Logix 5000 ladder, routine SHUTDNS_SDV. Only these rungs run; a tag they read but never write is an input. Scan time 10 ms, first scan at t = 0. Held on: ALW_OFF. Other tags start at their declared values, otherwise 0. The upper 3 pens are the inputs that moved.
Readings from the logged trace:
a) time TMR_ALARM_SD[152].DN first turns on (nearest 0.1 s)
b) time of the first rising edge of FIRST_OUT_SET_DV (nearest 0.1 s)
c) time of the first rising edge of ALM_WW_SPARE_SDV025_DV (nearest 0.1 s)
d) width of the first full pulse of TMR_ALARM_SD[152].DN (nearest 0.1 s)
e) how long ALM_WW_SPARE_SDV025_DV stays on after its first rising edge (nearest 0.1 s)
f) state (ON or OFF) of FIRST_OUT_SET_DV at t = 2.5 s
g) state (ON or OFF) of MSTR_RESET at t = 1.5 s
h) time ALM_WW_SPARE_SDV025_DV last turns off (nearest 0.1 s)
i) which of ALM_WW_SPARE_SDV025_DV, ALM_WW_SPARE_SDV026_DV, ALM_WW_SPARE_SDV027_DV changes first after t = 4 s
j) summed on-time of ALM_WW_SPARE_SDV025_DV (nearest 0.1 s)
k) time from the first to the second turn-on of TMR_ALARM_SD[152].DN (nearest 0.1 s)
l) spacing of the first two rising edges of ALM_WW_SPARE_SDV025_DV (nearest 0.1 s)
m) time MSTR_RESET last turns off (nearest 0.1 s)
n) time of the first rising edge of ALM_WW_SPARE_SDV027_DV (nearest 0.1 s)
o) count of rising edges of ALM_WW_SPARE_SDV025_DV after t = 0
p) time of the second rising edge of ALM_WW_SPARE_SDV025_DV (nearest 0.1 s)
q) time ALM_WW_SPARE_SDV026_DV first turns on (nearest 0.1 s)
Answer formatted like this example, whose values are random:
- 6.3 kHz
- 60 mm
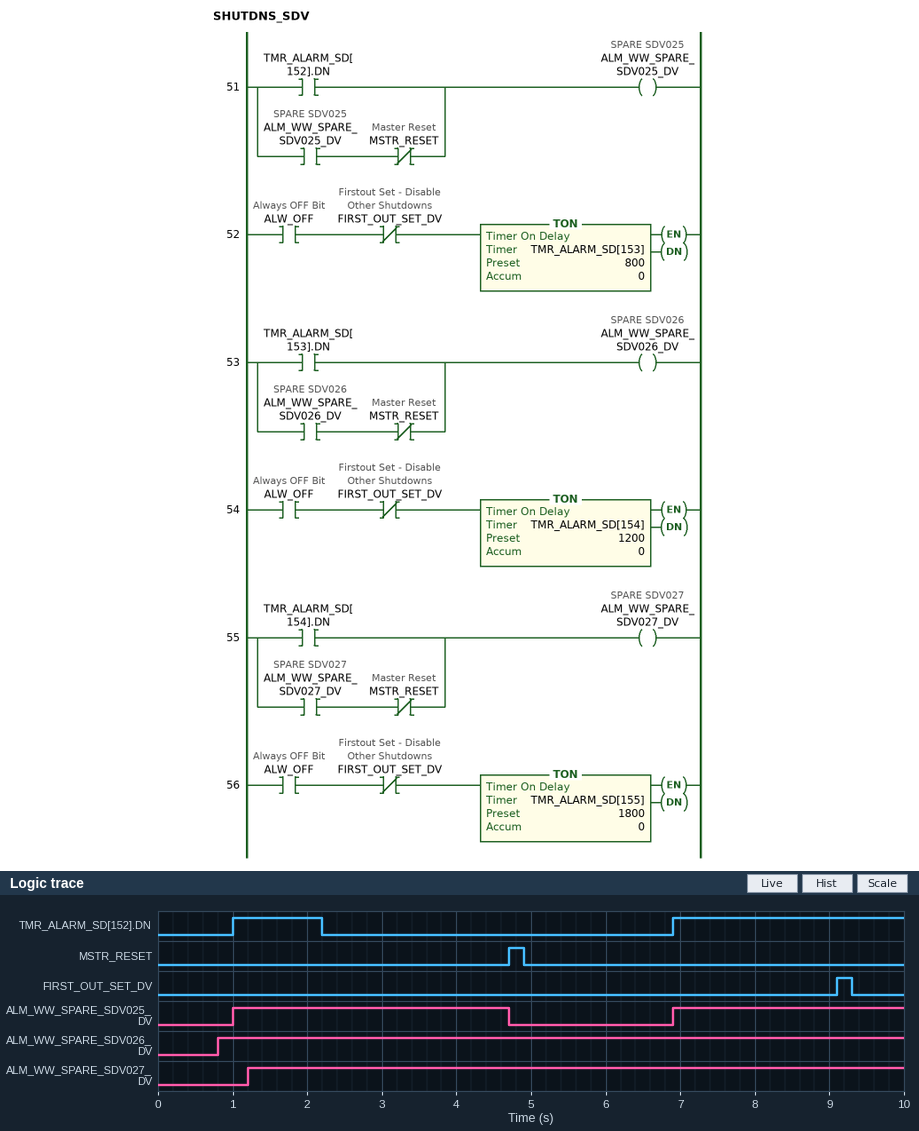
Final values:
- 1.0 s
- 9.1 s
- 1.0 s
- 1.2 s
- 3.7 s
- OFF
- OFF
- 4.7 s
- ALM_WW_SPARE_SDV025_DV
- 6.8 s
- 5.9 s
- 5.9 s
- 4.9 s
- 1.2 s
- 2
- 6.9 s
- 0.8 s
